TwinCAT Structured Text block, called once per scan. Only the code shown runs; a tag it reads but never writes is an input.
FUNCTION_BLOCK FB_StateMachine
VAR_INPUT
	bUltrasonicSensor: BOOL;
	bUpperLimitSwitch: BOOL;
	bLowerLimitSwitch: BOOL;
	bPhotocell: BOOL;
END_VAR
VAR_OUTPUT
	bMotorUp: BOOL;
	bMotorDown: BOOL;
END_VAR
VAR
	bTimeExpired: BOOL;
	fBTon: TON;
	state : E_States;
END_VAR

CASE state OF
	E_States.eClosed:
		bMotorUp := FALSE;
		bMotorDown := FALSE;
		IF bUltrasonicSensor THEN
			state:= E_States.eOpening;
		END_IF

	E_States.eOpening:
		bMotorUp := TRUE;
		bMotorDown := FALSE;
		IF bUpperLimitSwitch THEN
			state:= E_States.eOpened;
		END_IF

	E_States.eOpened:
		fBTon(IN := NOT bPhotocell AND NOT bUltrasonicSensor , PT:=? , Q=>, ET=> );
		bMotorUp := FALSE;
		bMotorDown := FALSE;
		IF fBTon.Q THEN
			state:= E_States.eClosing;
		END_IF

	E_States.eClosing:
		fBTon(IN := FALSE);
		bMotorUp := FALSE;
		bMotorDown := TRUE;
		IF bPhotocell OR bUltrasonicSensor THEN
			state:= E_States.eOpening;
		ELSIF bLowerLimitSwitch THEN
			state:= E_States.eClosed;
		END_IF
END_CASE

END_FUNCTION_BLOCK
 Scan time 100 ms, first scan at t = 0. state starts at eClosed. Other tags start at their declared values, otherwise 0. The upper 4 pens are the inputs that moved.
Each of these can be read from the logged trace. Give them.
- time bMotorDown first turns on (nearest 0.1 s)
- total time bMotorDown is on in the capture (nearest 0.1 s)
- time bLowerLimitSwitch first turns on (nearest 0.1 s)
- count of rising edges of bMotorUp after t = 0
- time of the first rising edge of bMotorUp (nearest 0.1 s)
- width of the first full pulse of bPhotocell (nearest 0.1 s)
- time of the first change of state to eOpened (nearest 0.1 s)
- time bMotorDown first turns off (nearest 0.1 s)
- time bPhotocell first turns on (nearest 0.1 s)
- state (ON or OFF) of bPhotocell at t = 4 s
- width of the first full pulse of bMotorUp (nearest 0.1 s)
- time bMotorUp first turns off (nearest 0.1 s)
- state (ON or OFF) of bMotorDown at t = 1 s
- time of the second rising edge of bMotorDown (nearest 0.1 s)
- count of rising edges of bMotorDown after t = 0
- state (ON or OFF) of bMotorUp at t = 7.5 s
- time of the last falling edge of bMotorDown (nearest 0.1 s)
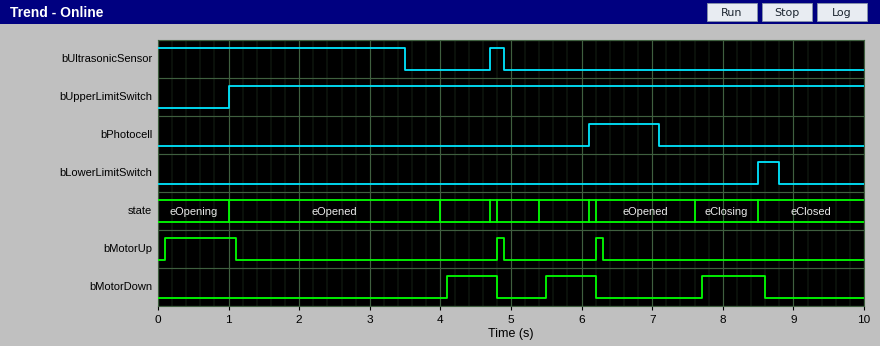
4.1 s
2.3 s
8.5 s
3
0.1 s
1.0 s
1.0 s
4.8 s
6.1 s
OFF
1.0 s
1.1 s
OFF
5.5 s
3
OFF
8.6 s
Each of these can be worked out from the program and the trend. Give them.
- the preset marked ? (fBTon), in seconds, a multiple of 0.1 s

0.5 s
